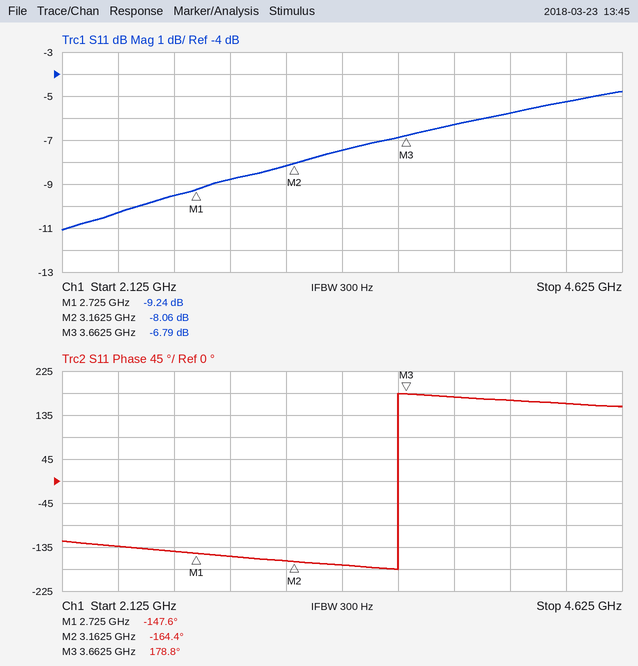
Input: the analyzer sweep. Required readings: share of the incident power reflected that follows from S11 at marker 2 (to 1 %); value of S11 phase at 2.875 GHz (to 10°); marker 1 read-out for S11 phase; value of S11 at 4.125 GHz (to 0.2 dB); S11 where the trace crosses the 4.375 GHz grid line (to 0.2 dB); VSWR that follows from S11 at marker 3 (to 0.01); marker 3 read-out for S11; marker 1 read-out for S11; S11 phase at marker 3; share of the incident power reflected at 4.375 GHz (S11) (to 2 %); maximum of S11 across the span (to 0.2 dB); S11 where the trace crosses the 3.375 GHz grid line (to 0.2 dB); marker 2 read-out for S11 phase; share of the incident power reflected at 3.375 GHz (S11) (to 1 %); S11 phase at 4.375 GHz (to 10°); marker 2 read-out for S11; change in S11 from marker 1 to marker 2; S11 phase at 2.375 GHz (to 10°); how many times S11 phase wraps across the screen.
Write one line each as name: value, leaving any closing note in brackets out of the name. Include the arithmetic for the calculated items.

share of the incident power reflected that follows from S11 at marker 2: 10^(-8.06/10) ≈ 16 %
value of S11 phase at 2.875 GHz: -150°
marker 1 read-out for S11 phase: -147.6°
value of S11 at 4.125 GHz: -5.8 dB
S11 where the trace crosses the 4.375 GHz grid line: -5.2 dB
VSWR that follows from S11 at marker 3: (1 + 0.4576)/(1 − 0.4576) ≈ 2.69
marker 3 read-out for S11: -6.79 dB
marker 1 read-out for S11: -9.24 dB
S11 phase at marker 3: 178.8°
share of the incident power reflected at 4.375 GHz (S11): 10^(-5.2/10) ≈ 30 %
maximum of S11 across the span: -4.8 dB
S11 where the trace crosses the 3.375 GHz grid line: -7.4 dB
marker 2 read-out for S11 phase: -164.4°
share of the incident power reflected at 3.375 GHz (S11): 10^(-7.4/10) ≈ 18 %
S11 phase at 4.375 GHz: 160°
marker 2 read-out for S11: -8.06 dB
change in S11 from marker 1 to marker 2: -8.06 − (-9.24) = 1.18 dB
S11 phase at 2.375 GHz: -130°
how many times S11 phase wraps across the screen: 1
